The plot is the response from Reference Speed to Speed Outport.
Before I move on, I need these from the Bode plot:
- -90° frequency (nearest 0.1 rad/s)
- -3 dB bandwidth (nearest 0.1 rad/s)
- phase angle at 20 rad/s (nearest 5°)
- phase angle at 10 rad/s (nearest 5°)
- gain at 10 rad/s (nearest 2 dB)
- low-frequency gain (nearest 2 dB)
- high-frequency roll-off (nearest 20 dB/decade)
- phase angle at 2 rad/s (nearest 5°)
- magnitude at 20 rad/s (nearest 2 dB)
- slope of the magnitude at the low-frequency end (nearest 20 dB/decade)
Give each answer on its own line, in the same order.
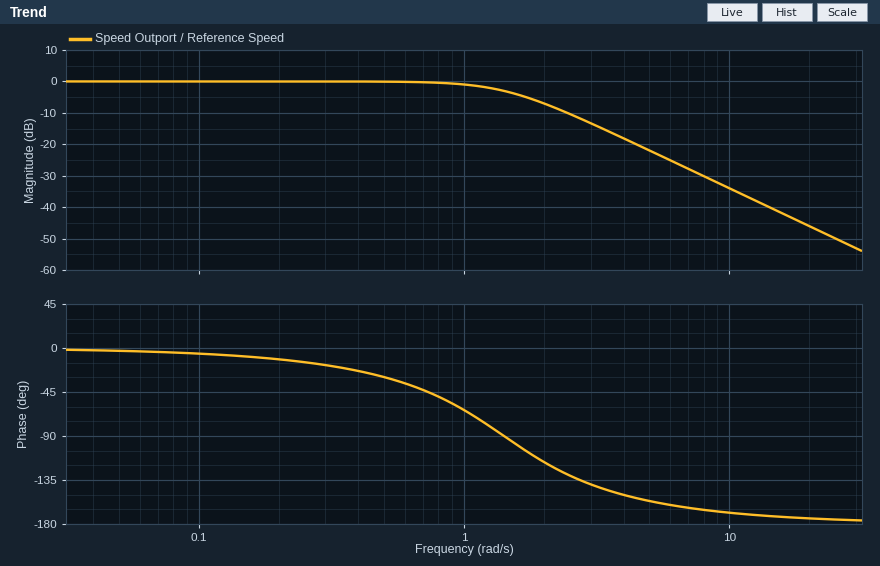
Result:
1.4 rad/s
1.4 rad/s
-175°
-170°
-34 dB
0 dB
-40 dB/decade
-115°
-46 dB
0 dB/decade
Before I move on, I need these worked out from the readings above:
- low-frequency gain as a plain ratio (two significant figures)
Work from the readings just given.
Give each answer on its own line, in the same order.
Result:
1.0
